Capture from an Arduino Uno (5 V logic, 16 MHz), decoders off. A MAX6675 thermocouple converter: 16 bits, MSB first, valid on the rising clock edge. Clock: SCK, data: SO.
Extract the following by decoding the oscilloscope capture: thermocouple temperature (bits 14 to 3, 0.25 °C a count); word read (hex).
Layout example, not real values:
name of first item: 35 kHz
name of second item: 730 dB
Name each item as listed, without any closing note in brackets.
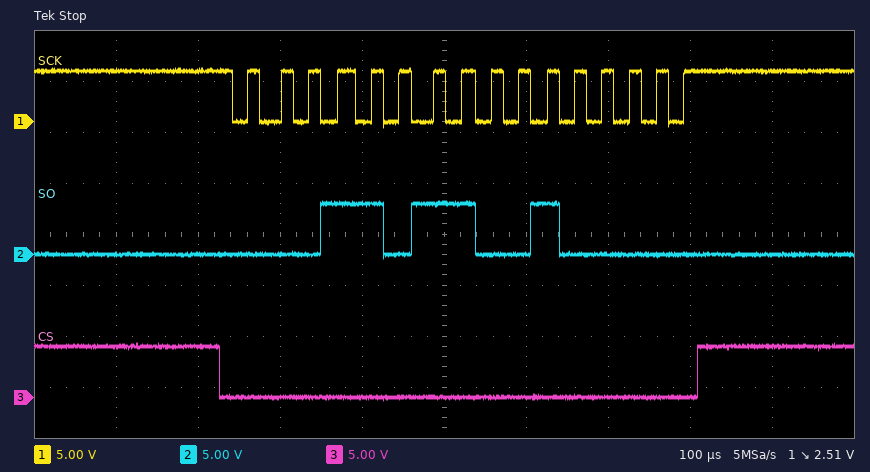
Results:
thermocouple temperature: 217.00 °C
word read: 0x1B20
